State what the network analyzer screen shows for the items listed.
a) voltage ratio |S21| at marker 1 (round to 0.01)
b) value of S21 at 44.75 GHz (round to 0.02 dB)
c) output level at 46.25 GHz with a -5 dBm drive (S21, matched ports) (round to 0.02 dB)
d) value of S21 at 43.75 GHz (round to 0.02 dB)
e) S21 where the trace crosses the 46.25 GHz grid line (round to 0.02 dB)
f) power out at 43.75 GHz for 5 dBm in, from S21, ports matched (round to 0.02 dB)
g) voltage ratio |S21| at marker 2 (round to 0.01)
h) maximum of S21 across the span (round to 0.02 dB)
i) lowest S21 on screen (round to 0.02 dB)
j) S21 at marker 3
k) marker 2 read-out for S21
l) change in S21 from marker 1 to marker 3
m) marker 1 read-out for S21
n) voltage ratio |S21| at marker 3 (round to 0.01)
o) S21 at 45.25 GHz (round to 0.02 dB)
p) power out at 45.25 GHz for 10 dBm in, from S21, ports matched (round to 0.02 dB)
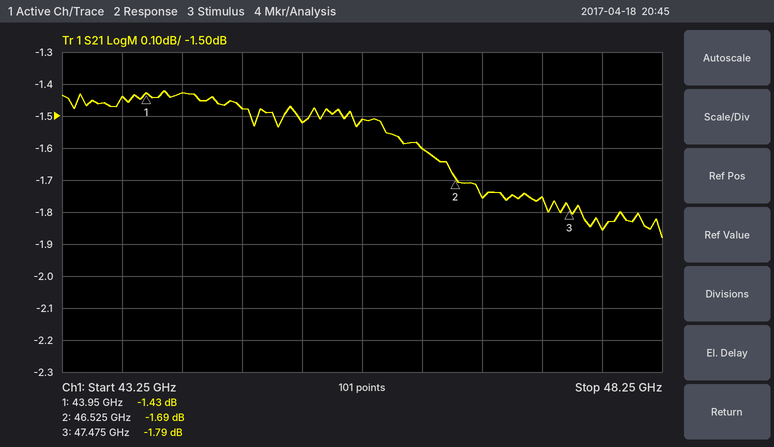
0.85
-1.48 dB
-6.60 dBm
-1.44 dB
-1.60 dB
3.56 dBm
0.82
-1.42 dB
-1.88 dB
-1.79 dB
-1.69 dB
-0.36 dB
-1.43 dB
0.81
-1.52 dB
8.48 dBm
